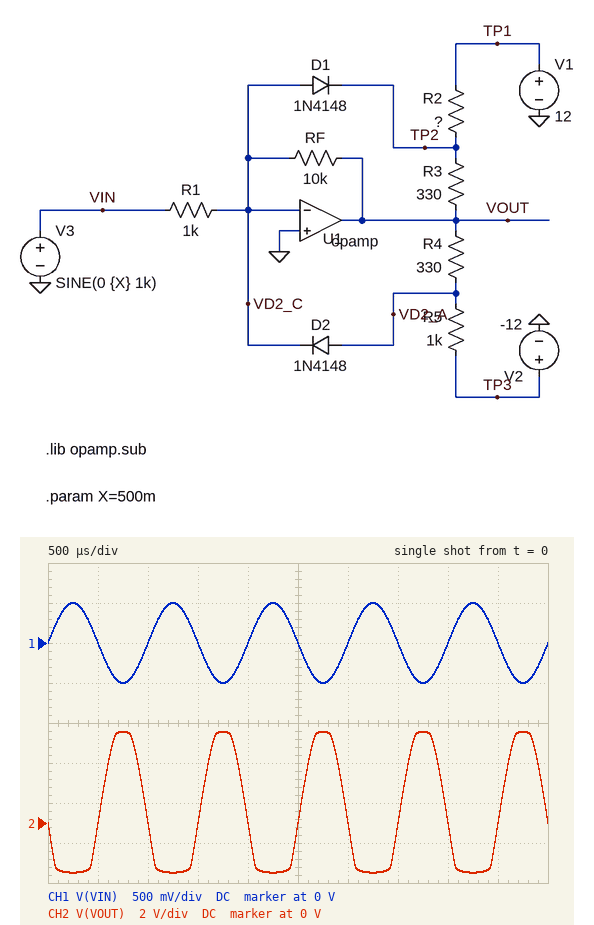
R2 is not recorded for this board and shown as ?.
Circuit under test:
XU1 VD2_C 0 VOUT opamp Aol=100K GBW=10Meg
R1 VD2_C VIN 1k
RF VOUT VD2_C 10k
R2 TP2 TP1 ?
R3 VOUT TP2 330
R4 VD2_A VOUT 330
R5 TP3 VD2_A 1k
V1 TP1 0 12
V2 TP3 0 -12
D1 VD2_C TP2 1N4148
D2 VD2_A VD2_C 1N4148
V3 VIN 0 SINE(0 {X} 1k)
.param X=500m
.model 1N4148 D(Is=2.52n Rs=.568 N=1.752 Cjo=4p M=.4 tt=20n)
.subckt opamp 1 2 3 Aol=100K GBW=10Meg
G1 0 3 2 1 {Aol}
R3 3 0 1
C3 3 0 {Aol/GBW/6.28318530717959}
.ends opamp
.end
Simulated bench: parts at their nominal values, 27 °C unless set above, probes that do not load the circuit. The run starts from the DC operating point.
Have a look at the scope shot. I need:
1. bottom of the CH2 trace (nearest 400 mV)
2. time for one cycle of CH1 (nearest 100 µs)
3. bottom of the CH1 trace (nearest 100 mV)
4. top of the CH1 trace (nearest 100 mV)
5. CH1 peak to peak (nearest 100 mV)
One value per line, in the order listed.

-2.4 V
1.0 ms
-500 mV
500 mV
1.0 V
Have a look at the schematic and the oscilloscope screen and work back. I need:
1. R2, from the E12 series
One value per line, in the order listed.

2.2 kΩ
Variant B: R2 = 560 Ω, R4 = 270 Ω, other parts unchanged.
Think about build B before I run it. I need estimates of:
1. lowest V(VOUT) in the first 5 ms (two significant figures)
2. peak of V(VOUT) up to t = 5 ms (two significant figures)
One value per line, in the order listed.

-5.0 V
3.9 V
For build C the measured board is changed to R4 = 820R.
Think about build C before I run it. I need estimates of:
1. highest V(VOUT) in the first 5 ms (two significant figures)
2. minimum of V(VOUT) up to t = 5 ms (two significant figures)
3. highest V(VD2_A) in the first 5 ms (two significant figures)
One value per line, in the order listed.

5.0 V
-2.5 V
-2.7 V
